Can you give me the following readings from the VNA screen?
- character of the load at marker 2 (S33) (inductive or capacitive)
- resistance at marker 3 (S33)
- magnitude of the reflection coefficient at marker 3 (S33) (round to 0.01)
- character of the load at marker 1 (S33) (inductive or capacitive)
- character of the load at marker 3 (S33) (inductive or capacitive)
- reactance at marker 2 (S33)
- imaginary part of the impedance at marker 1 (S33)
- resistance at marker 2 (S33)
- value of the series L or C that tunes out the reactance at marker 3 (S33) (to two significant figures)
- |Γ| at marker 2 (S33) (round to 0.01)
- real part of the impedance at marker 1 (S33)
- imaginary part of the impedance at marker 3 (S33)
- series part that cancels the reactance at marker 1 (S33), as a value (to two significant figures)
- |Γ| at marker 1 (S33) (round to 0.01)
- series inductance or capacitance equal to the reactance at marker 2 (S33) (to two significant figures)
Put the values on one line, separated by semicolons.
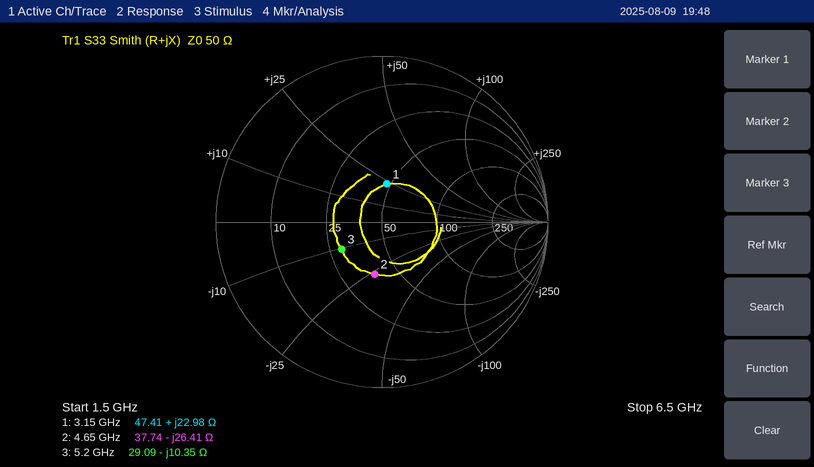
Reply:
capacitive; 29.09 Ω; 0.29; inductive; capacitive; -26.41 Ω; +22.98 Ω; 37.74 Ω; 320 pH; 0.32; 47.41 Ω; -10.35 Ω; 2.2 pF; 0.23; 1.3 pF
